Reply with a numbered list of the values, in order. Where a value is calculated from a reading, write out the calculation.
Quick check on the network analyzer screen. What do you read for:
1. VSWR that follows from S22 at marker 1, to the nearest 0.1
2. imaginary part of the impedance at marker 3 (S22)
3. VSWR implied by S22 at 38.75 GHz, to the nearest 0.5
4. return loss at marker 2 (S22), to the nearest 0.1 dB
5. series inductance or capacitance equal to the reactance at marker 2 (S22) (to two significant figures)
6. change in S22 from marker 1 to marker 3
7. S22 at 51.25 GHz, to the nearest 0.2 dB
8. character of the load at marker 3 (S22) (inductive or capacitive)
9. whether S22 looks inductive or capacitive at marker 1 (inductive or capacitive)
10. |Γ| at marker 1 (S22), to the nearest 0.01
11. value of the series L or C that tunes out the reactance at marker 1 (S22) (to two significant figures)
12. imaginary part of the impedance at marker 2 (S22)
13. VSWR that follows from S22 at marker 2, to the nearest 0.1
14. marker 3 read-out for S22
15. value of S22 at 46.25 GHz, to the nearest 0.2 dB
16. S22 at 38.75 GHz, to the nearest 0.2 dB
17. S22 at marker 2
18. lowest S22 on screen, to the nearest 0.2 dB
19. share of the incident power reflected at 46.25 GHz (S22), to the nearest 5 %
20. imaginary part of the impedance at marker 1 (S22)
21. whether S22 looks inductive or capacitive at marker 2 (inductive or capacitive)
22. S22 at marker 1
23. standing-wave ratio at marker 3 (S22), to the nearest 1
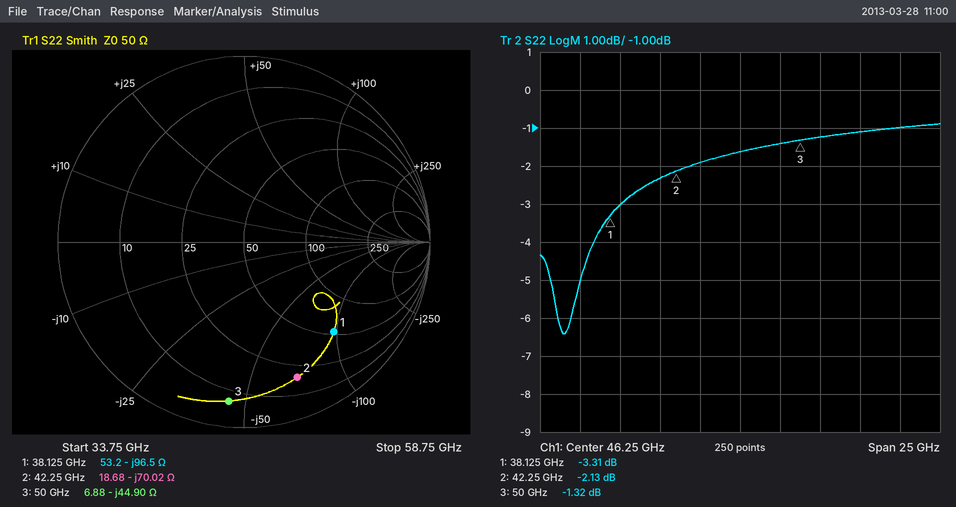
1. (1 + 0.6831)/(1 − 0.6831) ≈ 5.3
2. -44.90 Ω
3. |Γ| = 10^(-3/20) = 0.7079; VSWR = (1 + 0.7079)/(1 − 0.7079) ≈ 5.85, so 6.0 to the nearest 0.5
4. 2.1 dB
5. C = 1/(2π × 42.25 GHz × 70.02 Ω) ≈ 54 fF
6. -1.32 − (-3.31) = 1.99 dB
7. -1.2 dB
8. capacitive
9. capacitive
10. 0.68
11. L = 96.5 Ω/(2π × 38.125 GHz) ≈ 403 pH, so 400 pH to two significant figures
12. -70.02 Ω
13. (1 + 0.7825)/(1 − 0.7825) ≈ 8.2
14. -1.32 dB
15. -1.6 dB
16. -3.0 dB
17. -2.13 dB
18. -6.4 dB
19. 10^(-1.6/10) ≈ 69.2 %, so 70 % to the nearest 5 %
20. -96.5 Ω
21. capacitive
22. -3.31 dB
23. 13
